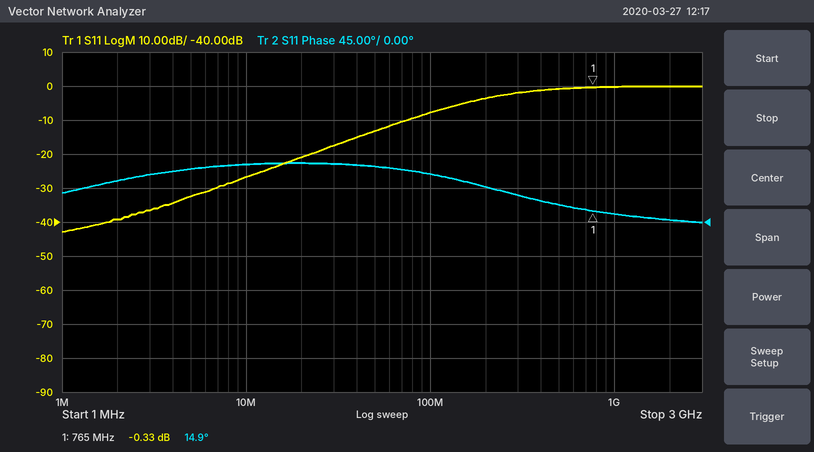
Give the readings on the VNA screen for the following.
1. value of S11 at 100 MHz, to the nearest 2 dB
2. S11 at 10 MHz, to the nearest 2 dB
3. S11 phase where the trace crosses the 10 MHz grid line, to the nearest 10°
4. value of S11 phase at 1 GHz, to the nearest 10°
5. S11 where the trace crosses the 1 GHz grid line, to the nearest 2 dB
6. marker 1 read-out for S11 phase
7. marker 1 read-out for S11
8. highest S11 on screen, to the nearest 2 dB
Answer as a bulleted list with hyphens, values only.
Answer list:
- -8 dB
- -26 dB
- 80°
- 10°
- 0 dB
- 14.9°
- -0.33 dB
- 0 dB
